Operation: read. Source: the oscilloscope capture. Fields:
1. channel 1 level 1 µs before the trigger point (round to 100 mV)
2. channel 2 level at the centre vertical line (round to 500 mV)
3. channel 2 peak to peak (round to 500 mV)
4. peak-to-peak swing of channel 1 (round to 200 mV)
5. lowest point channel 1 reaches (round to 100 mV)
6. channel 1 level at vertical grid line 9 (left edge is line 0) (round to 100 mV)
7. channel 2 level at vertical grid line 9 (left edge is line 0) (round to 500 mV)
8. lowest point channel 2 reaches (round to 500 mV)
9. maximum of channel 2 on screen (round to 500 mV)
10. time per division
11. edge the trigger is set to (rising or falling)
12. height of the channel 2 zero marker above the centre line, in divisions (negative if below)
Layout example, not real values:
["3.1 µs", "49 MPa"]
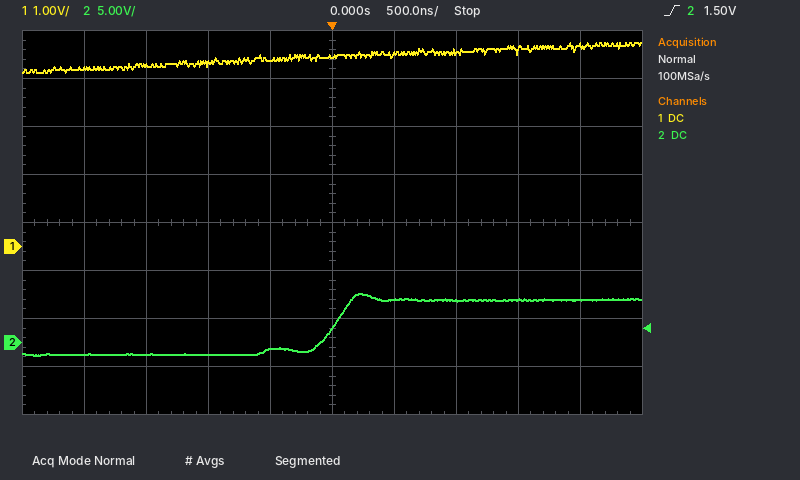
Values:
["3.8 V", "1.5 V", "6.5 V", "600 mV", "3.6 V", "4.2 V", "4.5 V", "-1.5 V", "5.0 V", "500 ns", "rising", "-2.5 div"]
